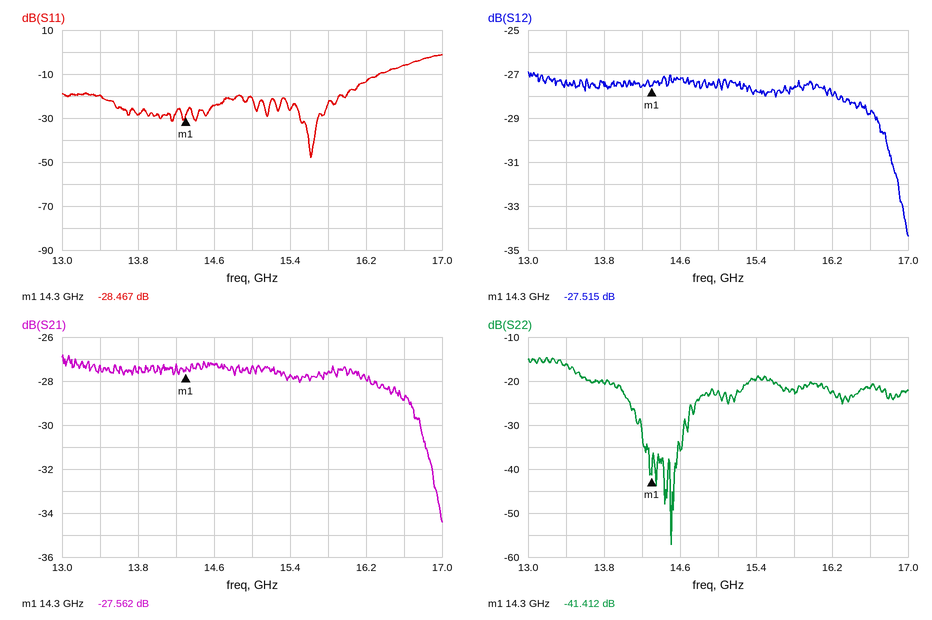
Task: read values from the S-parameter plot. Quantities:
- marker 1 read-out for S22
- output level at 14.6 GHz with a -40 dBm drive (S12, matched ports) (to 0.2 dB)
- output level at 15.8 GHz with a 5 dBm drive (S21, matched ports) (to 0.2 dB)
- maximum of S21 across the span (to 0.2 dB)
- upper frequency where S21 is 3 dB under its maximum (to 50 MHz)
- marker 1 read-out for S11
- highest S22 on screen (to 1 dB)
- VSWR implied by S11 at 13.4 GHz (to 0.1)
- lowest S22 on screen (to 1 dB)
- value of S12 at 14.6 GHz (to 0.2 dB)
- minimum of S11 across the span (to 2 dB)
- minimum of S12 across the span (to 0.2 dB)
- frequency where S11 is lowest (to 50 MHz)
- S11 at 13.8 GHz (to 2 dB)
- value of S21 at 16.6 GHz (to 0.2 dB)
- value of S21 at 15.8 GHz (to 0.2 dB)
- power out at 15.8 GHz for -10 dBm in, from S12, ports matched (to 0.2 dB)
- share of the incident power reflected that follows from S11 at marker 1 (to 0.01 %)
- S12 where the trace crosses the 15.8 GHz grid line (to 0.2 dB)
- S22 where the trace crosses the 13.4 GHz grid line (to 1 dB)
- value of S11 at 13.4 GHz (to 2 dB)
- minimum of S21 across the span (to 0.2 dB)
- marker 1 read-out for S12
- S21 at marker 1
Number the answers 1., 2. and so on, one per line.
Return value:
1. -41.412 dB
2. -67.2 dBm
3. -22.6 dBm
4. -26.8 dB
5. 16.75 GHz
6. -28.467 dB
7. -15 dB
8. 1.2
9. -57 dB
10. -27.2 dB
11. -48 dB
12. -34.4 dB
13. 15.60 GHz
14. -28 dB
15. -28.8 dB
16. -27.6 dB
17. -37.6 dBm
18. 0.14 %
19. -27.6 dB
20. -16 dB
21. -20 dB
22. -34.4 dB
23. -27.515 dB
24. -27.562 dB
